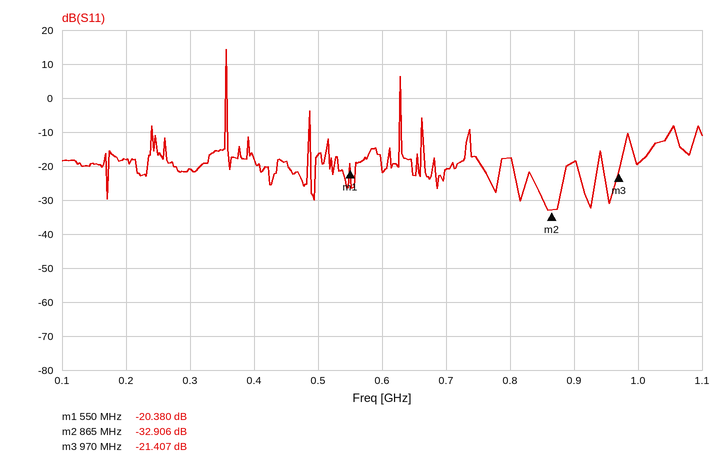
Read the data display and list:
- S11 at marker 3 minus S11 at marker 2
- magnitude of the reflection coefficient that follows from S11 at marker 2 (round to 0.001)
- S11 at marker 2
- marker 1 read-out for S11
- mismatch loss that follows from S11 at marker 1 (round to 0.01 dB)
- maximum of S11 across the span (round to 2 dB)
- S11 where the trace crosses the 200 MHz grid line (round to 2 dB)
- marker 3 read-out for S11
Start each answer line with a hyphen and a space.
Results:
- 11.499 dB
- 0.023
- -32.906 dB
- -20.380 dB
- 0.04 dB
- 14 dB
- -18 dB
- -21.407 dB
